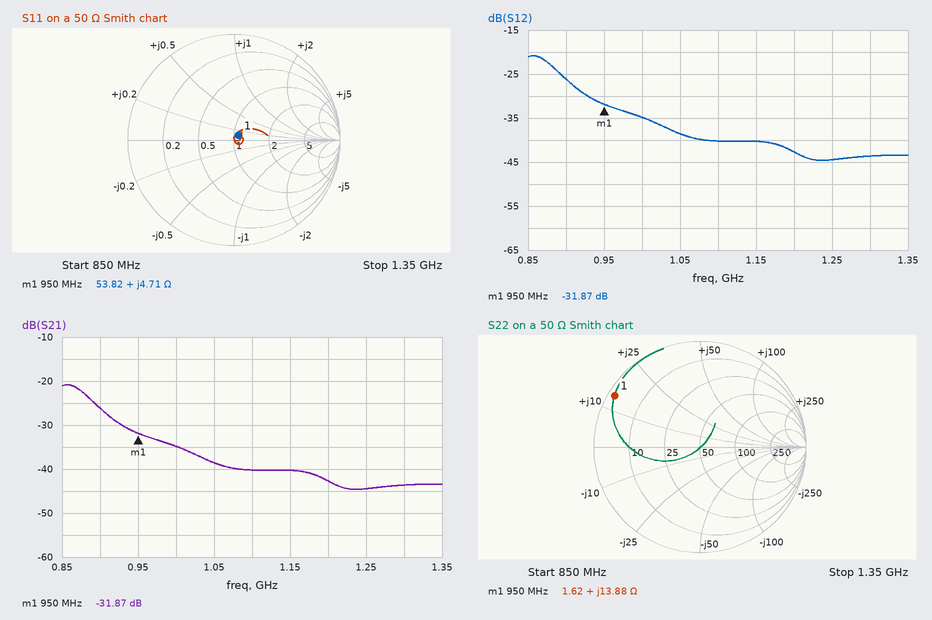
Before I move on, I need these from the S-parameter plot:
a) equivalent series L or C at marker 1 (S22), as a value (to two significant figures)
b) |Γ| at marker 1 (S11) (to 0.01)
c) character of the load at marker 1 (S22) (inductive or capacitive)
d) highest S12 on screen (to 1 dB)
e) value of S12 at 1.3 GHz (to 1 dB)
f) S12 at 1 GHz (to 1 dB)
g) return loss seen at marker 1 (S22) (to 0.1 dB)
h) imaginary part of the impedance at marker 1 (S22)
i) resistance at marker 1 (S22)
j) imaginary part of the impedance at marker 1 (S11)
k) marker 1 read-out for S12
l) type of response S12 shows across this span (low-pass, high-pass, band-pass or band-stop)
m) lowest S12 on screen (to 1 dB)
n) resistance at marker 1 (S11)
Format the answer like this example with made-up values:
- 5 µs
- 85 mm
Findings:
- 2.3 nH
- 0.06
- inductive
- -21 dB
- -44 dB
- -35 dB
- 0.5 dB
- +13.88 Ω
- 1.62 Ω
- +4.71 Ω
- -31.87 dB
- low-pass
- -45 dB
- 53.82 Ω
